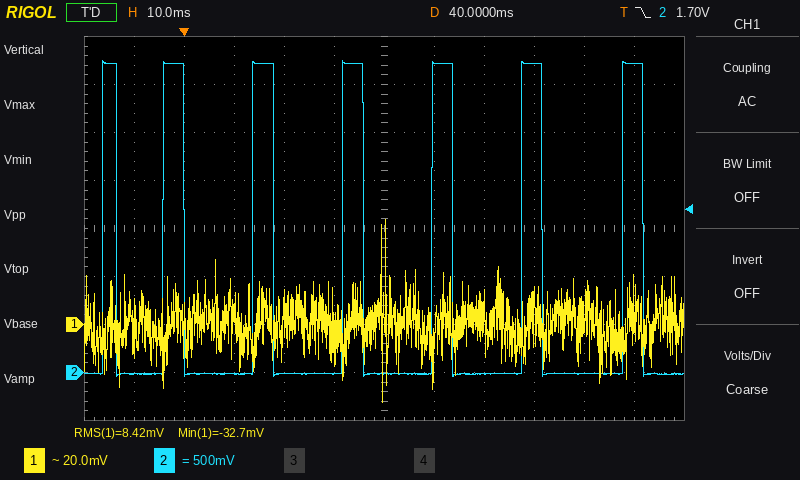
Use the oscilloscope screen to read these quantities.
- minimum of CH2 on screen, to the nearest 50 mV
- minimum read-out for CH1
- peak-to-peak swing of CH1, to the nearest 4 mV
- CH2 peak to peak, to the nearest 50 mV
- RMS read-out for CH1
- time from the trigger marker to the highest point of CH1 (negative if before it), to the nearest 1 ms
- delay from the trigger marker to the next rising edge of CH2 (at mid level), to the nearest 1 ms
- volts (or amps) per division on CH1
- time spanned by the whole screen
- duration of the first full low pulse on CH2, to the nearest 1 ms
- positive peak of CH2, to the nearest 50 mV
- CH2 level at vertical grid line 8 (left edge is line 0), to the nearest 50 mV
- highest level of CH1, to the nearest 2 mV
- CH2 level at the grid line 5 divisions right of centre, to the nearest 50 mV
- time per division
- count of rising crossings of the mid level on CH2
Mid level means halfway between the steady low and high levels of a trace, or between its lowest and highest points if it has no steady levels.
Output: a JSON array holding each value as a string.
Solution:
["-50 mV", "-32.7 mV", "76 mV", "3.30 V", "8.42 mV", "+40 ms", "14 ms", "20 mV", "120 ms", "9 ms", "3.25 V", "0 mV", "44 mV", "3.20 V", "10 ms", "7"]
